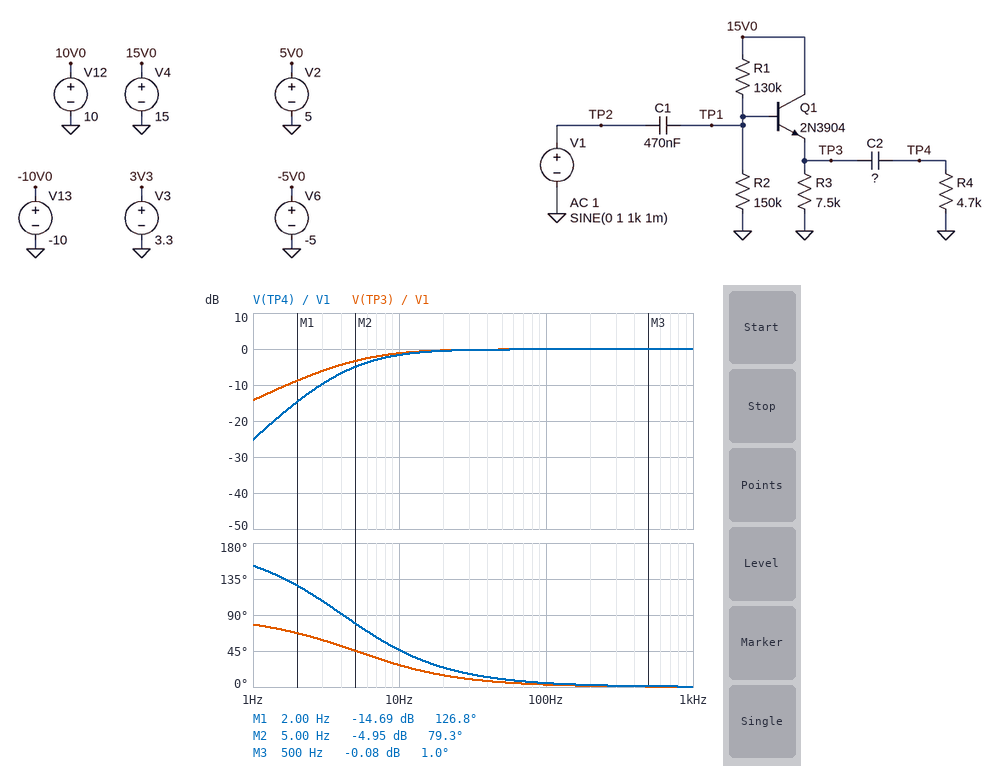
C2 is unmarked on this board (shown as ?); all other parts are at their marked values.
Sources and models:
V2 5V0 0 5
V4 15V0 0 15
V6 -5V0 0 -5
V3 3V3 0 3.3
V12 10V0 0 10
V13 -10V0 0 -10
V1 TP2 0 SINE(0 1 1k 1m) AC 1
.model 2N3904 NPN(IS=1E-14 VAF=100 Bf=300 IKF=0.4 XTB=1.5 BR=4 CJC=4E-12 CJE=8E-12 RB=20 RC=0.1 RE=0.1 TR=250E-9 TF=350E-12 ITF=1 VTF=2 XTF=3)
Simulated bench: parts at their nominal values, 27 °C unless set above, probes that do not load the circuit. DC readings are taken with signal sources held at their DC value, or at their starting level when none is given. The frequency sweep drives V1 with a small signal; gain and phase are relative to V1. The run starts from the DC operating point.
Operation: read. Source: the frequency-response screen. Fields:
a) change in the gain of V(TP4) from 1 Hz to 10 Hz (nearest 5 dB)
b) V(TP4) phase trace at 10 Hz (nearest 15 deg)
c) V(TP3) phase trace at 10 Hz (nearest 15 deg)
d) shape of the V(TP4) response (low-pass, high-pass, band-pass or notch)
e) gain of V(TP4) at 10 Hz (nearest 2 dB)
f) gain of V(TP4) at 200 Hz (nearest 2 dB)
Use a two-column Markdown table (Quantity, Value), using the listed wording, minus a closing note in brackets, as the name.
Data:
| Quantity | Value |
|---|---|
| change in the gain of V(TP4) from 1 Hz to 10 Hz | 25 dB |
| V(TP4) phase trace at 10 Hz | 45 deg |
| V(TP3) phase trace at 10 Hz | 30 deg |
| shape of the V(TP4) response | high-pass |
| gain of V(TP4) at 10 Hz | -2 dB |
| gain of V(TP4) at 200 Hz | 0 dB |
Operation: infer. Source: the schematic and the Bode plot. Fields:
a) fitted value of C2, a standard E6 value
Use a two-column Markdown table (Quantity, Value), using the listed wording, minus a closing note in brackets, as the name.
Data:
| Quantity | Value |
|---|---|
| fitted value of C2, a standard E6 value | 10 µF |
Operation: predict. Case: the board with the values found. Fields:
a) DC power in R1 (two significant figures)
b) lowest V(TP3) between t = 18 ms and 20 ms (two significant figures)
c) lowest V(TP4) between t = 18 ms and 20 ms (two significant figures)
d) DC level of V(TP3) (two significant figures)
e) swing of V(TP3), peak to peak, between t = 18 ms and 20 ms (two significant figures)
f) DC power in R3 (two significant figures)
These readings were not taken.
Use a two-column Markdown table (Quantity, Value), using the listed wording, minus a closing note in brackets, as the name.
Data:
| Quantity | Value |
|---|---|
| DC power in R1 | 400 µW |
| lowest V(TP3) between t = 18 ms and 20 ms | 6.2 V |
| lowest V(TP4) between t = 18 ms and 20 ms | -990 mV |
| DC level of V(TP3) | 7.2 V |
| swing of V(TP3), peak to peak, between t = 18 ms and 20 ms | 2.0 V |
| DC power in R3 | 6.9 mW |
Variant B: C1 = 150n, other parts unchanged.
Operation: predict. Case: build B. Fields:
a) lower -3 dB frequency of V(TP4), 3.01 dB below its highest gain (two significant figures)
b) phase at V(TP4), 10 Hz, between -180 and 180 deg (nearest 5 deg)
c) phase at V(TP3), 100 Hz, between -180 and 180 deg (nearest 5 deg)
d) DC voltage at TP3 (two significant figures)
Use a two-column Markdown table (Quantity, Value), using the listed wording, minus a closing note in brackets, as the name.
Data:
| Quantity | Value |
|---|---|
| lower -3 dB frequency of V(TP4), 3.01 dB below its highest gain | 17 Hz |
| phase at V(TP4), 10 Hz, between -180 and 180 deg | 75 deg |
| phase at V(TP3), 100 Hz, between -180 and 180 deg | 10 deg |
| DC voltage at TP3 | 7.2 V |
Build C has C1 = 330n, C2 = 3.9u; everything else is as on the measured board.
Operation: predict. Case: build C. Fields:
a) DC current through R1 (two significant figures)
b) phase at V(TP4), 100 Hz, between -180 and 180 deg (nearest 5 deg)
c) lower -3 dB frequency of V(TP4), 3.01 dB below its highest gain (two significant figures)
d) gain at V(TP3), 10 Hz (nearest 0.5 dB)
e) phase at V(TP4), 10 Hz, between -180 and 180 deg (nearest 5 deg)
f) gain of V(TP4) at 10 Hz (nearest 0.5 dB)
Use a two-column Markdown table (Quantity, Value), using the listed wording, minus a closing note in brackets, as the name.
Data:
| Quantity | Value |
|---|---|
| DC current through R1 | 55 µA |
| phase at V(TP4), 100 Hz, between -180 and 180 deg | 10 deg |
| lower -3 dB frequency of V(TP4), 3.01 dB below its highest gain | 13 Hz |
| gain at V(TP3), 10 Hz | -2.0 dB |
| phase at V(TP4), 10 Hz, between -180 and 180 deg | 75 deg |
| gain of V(TP4) at 10 Hz | -4.5 dB |
